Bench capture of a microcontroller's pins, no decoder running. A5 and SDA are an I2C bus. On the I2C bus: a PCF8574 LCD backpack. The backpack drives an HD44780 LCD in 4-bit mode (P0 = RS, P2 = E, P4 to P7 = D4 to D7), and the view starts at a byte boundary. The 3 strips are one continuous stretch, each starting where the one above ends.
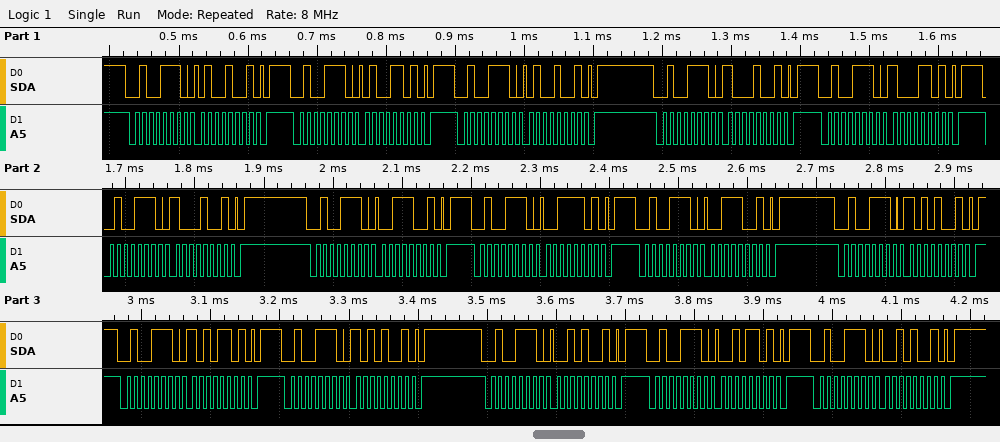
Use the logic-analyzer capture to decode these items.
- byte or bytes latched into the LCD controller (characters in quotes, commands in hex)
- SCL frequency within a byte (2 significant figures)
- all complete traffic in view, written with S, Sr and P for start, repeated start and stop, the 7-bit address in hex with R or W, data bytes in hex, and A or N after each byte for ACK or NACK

'H' ':'
100 kHz
S 27W A 49 A P S 27W A 4D A P S 27W A 49 A P S 27W A 89 A P S 27W A 8D A P S 27W A 89 A P S 27W A 39 A P S 27W A 3D A P S 27W A 39 A P S 27W A A9 A P S 27W A AD A P S 27W A A9 A P S 27W A 29 A P S 27W A 2D A P S 27W A 29 A P
